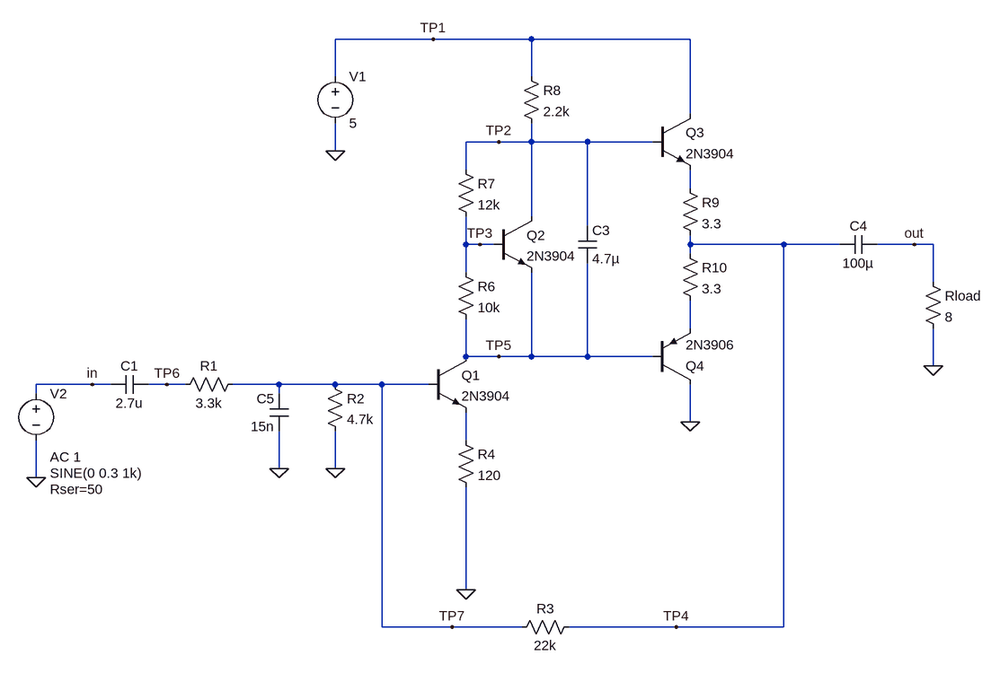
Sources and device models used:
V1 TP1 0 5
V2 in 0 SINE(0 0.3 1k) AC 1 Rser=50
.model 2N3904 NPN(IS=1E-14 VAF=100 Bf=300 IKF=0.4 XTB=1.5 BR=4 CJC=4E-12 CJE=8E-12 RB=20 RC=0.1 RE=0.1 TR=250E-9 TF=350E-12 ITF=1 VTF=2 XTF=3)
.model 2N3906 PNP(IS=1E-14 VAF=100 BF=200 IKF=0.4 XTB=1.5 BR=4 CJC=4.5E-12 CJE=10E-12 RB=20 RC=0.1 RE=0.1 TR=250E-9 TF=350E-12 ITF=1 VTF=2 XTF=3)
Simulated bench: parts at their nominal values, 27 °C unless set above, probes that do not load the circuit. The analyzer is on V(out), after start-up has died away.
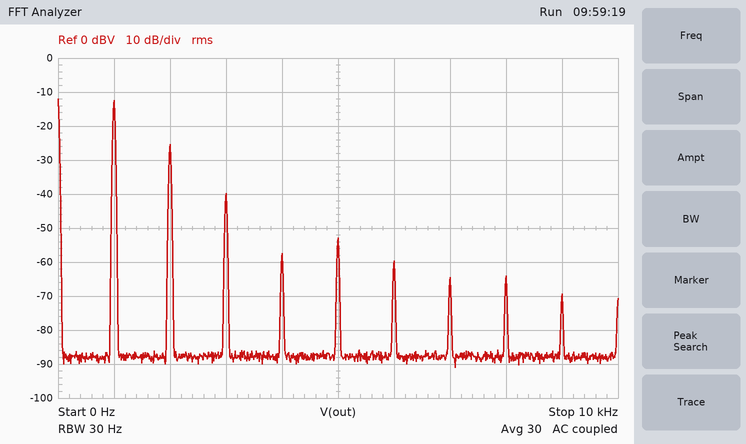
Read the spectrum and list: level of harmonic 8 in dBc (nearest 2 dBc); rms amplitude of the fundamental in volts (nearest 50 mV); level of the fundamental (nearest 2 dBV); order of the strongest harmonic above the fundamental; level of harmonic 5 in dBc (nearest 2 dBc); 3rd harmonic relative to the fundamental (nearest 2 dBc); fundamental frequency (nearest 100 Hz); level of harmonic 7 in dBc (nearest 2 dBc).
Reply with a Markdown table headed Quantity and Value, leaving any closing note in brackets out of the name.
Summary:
| Quantity | Value |
|---|---|
| level of harmonic 8 in dBc | -52 dBc |
| rms amplitude of the fundamental in volts | 250 mV |
| level of the fundamental | -12 dBV |
| order of the strongest harmonic above the fundamental | 2 |
| level of harmonic 5 in dBc | -40 dBc |
| 3rd harmonic relative to the fundamental | -28 dBc |
| fundamental frequency | 1.0 kHz |
| level of harmonic 7 in dBc | -52 dBc |
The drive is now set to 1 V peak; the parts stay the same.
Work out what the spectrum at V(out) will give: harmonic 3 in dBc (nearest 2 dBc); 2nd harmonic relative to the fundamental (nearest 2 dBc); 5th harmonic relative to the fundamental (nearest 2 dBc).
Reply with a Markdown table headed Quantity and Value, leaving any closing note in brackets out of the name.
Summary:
| Quantity | Value |
|---|---|
| harmonic 3 in dBc | -30 dBc |
| 2nd harmonic relative to the fundamental | -6 dBc |
| 5th harmonic relative to the fundamental | -32 dBc |
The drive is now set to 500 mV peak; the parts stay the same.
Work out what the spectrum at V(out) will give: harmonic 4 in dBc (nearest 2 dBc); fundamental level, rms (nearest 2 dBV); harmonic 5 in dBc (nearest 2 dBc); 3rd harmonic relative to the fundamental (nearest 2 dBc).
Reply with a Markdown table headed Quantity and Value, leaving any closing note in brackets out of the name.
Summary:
| Quantity | Value |
|---|---|
| harmonic 4 in dBc | -26 dBc |
| fundamental level, rms | -10 dBV |
| harmonic 5 in dBc | -38 dBc |
| 3rd harmonic relative to the fundamental | -32 dBc |
